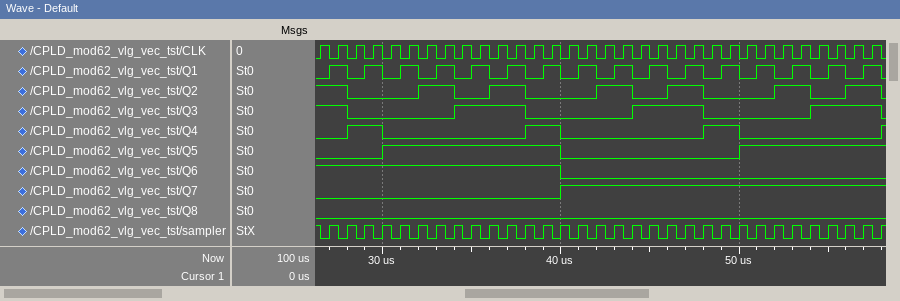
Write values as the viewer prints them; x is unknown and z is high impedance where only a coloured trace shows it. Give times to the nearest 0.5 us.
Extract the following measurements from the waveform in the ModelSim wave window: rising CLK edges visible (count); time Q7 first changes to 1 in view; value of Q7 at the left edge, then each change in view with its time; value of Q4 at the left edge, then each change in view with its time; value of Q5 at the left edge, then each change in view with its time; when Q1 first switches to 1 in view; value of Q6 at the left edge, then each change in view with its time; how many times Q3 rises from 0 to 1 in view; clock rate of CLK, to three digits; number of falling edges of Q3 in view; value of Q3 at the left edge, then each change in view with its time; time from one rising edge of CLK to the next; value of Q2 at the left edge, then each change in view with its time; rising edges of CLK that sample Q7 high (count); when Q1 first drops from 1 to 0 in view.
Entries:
32
40 us
0, 1 at 40 us
0, 1 at 28 us, 0 at 30 us, 1 at 38 us, 0 at 40 us, 1 at 48 us, 0 at 50 us, 1 at 58 us
0, 1 at 30 us, 0 at 40 us, 1 at 50 us
27 us
1, 0 at 40 us
3
1.00 MHz
4
1, 0 at 28 us, 1 at 34 us, 0 at 38 us, 1 at 44 us, 0 at 48 us, 1 at 54 us, 0 at 58 us
1 us
1, 0 at 28 us, 1 at 32 us, 0 at 34 us, 1 at 36 us, 0 at 38 us, 1 at 42 us, 0 at 44 us, 1 at 46 us, 0 at 48 us, 1 at 52 us, 0 at 54 us, 1 at 56 us, 0 at 58 us
18
28 us
